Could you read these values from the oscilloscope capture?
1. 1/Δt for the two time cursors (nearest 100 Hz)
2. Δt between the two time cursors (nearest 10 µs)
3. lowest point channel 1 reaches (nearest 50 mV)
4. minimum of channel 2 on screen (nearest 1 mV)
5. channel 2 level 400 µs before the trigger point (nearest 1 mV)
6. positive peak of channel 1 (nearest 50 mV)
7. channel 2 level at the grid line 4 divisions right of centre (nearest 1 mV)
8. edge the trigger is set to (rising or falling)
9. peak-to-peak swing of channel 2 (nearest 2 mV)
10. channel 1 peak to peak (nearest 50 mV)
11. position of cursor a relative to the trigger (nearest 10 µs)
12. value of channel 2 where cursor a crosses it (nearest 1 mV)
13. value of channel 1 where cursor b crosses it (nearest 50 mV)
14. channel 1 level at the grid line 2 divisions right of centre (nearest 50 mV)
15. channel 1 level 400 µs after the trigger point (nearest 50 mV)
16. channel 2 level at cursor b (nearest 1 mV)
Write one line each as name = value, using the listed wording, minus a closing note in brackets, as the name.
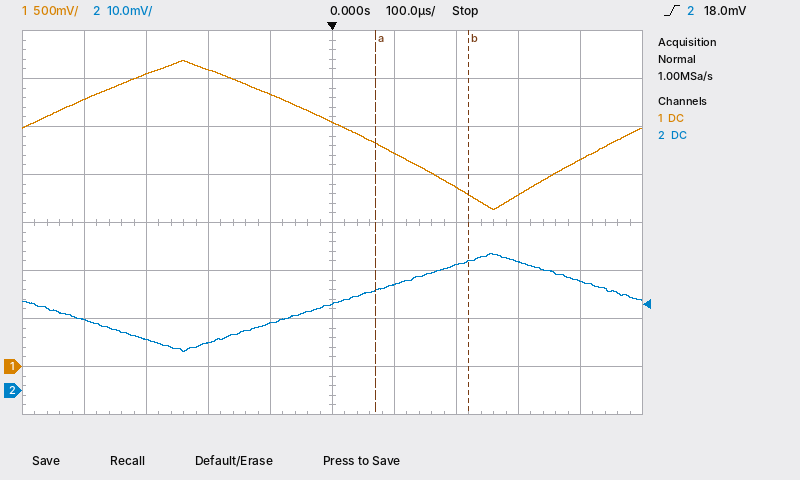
1/Δt for the two time cursors = 6.7 kHz
Δt between the two time cursors = 150 µs
lowest point channel 1 reaches = 1.65 V
minimum of channel 2 on screen = 8 mV
channel 2 level 400 µs before the trigger point = 15 mV
positive peak of channel 1 = 3.20 V
channel 2 level at the grid line 4 divisions right of centre = 23 mV
edge the trigger is set to = rising
peak-to-peak swing of channel 2 = 20 mV
channel 1 peak to peak = 1.55 V
position of cursor a relative to the trigger = +70 µs
value of channel 2 where cursor a crosses it = 21 mV
value of channel 1 where cursor b crosses it = 1.80 V
channel 1 level at the grid line 2 divisions right of centre = 1.85 V
channel 1 level 400 µs after the trigger point = 2.15 V
channel 2 level at cursor b = 27 mV
